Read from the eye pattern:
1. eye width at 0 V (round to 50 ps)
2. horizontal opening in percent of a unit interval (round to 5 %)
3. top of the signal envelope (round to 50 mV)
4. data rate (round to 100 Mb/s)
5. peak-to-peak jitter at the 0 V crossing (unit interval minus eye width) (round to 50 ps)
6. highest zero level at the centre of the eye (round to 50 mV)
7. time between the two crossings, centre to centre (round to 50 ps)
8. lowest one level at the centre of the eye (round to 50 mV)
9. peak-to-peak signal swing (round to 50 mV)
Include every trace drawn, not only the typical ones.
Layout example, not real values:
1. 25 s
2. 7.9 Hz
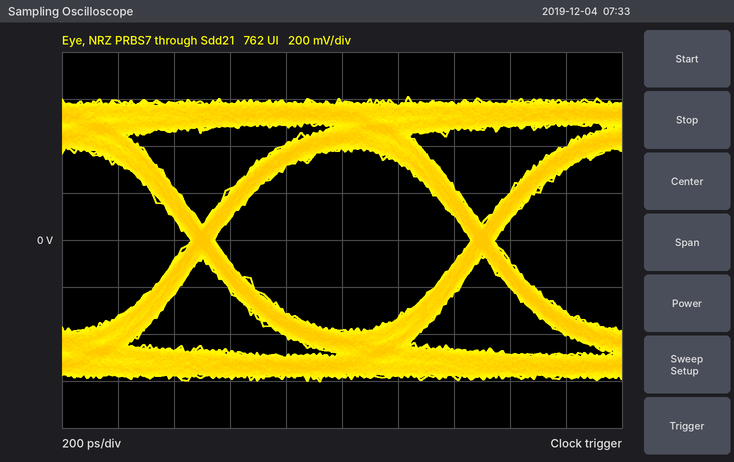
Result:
1. 900 ps
2. 90 %
3. 600 mV
4. 1.0 Gb/s
5. 100 ps
6. -400 mV
7. 1.00 ns
8. 400 mV
9. 1.20 V
